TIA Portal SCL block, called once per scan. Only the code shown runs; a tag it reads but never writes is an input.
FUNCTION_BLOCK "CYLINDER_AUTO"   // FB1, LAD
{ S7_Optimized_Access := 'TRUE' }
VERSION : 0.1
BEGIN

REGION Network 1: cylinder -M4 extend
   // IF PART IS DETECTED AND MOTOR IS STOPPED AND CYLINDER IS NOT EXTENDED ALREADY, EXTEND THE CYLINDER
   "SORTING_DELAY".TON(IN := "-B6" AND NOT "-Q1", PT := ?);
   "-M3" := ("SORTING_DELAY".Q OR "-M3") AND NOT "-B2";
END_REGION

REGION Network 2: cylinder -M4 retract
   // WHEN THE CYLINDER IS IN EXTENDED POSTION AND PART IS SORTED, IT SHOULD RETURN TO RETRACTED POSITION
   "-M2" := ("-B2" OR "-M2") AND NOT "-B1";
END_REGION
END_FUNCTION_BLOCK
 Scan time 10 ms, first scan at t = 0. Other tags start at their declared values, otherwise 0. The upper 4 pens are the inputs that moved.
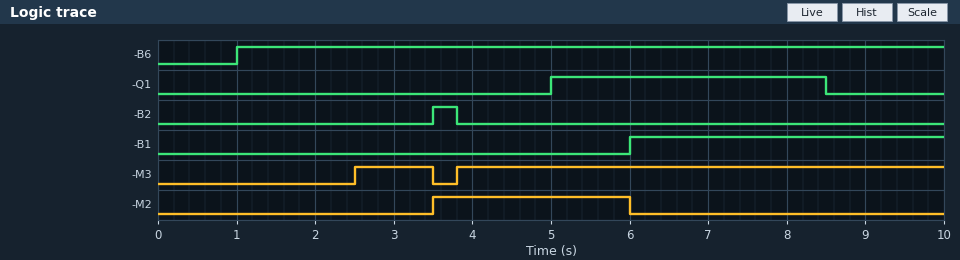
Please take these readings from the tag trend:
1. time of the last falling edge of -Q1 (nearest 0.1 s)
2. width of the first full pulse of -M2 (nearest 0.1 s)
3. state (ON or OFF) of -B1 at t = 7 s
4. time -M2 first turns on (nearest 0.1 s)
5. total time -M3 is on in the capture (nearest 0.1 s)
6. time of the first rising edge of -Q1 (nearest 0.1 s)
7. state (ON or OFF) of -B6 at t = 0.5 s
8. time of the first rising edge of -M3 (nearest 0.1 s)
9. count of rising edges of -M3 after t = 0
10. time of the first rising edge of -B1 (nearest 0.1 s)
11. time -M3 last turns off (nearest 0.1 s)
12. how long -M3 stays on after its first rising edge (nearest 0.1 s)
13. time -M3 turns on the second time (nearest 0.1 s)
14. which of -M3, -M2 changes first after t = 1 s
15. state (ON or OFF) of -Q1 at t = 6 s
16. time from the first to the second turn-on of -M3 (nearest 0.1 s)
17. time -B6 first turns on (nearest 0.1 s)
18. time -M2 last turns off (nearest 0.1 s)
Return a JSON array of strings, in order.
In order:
["8.5 s", "2.5 s", "ON", "3.5 s", "7.2 s", "5.0 s", "OFF", "2.5 s", "2", "6.0 s", "3.5 s", "1.0 s", "3.8 s", "-M3", "ON", "1.3 s", "1.0 s", "6.0 s"]
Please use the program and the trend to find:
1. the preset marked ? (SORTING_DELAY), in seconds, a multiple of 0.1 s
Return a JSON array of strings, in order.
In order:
["1.5 s"]
